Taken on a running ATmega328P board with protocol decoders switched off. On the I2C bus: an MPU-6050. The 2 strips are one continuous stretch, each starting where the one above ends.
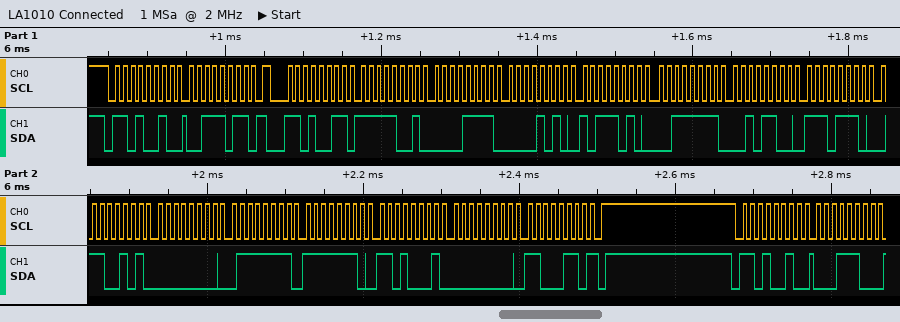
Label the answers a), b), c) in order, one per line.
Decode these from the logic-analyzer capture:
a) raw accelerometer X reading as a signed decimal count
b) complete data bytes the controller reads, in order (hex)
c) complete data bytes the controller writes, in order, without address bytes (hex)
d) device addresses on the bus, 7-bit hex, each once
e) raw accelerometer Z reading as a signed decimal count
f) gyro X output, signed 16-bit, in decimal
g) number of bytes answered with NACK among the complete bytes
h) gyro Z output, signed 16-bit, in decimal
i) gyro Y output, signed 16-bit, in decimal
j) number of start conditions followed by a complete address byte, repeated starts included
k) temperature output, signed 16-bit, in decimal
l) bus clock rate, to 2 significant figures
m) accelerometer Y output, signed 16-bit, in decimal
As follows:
a) -1777
b) F9 0F 0A BA 3F 2C EE 65 00 7F FE D1 00 C6
c) 3B 1C
d) 0x69
e) 16172
f) 127
g) 1
h) 198
i) -303
j) 3
k) -4507
l) 100 kHz
m) 2746
